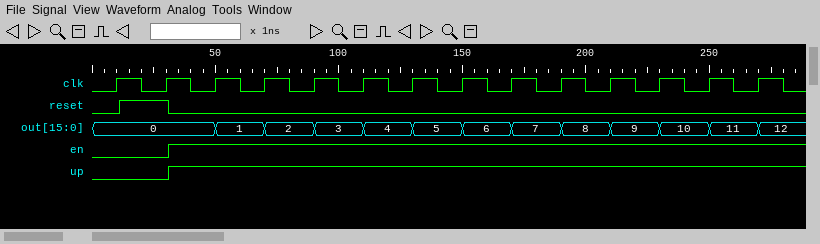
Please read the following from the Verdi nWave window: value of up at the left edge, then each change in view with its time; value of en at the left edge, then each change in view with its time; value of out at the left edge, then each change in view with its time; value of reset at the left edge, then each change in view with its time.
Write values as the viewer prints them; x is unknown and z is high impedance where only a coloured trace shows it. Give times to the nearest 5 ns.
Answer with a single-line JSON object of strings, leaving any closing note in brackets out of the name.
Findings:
{"value of up at the left edge, then each change in view with its time": "0, 1 at 30 ns", "value of en at the left edge, then each change in view with its time": "0, 1 at 30 ns", "value of out at the left edge, then each change in view with its time": "0, 1 at 50 ns, 2 at 70 ns, 3 at 90 ns, 4 at 110 ns, 5 at 130 ns, 6 at 150 ns, 7 at 170 ns, 8 at 190 ns, 9 at 210 ns, 10 at 230 ns, 11 at 250 ns, 12 at 270 ns", "value of reset at the left edge, then each change in view with its time": "0, 1 at 10 ns, 0 at 30 ns"}
